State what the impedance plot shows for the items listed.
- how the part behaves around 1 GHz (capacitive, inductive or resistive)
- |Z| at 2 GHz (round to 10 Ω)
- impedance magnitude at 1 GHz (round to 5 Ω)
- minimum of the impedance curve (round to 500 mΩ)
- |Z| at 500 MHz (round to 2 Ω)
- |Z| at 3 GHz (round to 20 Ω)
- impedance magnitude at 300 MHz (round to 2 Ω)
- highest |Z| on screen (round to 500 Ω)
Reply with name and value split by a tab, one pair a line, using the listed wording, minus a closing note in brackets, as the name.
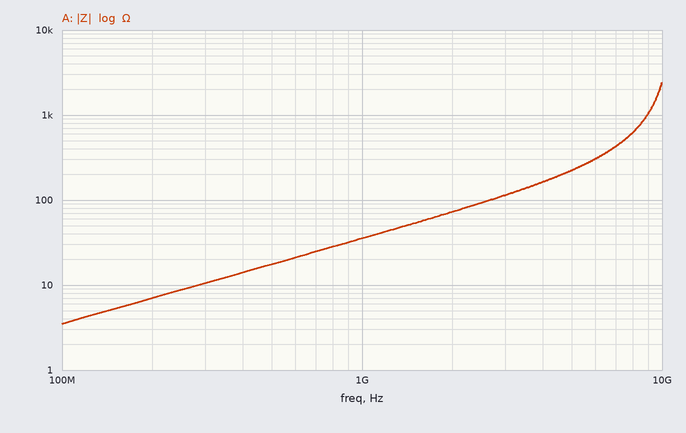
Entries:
how the part behaves around 1 GHz	inductive
|Z| at 2 GHz	70 Ω
impedance magnitude at 1 GHz	35 Ω
minimum of the impedance curve	3.5 Ω
|Z| at 500 MHz	18 Ω
|Z| at 3 GHz	120 Ω
impedance magnitude at 300 MHz	10 Ω
highest |Z| on screen	2.5 kΩ
